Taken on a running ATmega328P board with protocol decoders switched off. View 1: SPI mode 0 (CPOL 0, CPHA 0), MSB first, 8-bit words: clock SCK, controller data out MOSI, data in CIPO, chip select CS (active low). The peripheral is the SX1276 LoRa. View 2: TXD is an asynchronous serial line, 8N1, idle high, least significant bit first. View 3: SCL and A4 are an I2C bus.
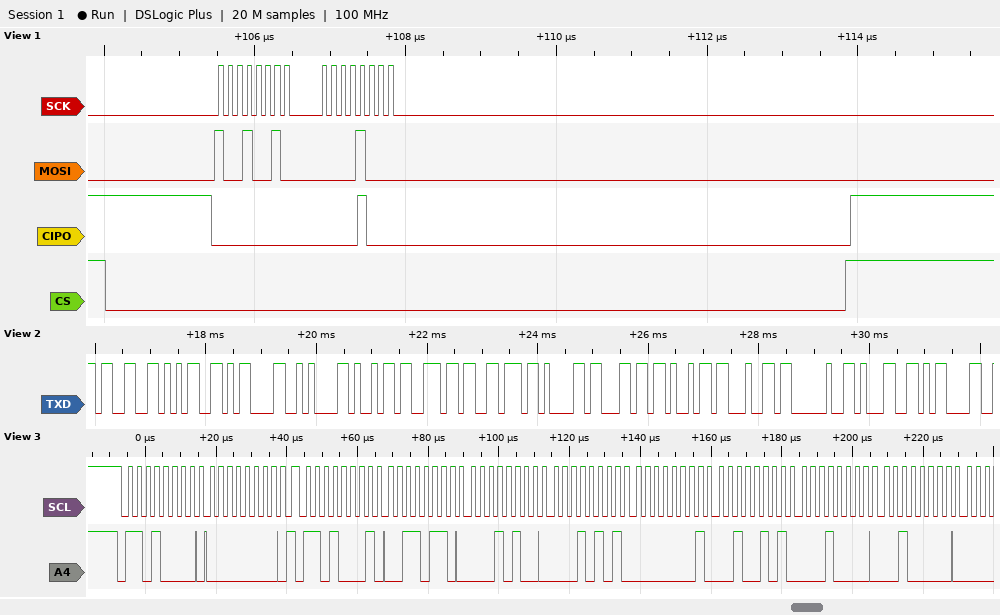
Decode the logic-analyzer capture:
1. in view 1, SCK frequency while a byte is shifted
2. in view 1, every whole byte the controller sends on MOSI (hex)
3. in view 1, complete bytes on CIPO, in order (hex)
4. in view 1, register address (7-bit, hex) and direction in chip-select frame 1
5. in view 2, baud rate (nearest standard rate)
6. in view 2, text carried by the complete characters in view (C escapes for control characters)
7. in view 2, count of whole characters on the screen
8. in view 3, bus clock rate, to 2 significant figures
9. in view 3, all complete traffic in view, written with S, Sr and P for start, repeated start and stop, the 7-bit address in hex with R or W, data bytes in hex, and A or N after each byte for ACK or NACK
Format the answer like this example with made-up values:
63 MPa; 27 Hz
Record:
8 MHz; 92 08; 00 08; 0x12 write; 9600 baud; "35\r\ninvalid 1\r"; 14; 400 kHz; S 68W A 00 A Sr 68R A 36 A 14 A 15 A 01 A 25 A 10 A 20 A
